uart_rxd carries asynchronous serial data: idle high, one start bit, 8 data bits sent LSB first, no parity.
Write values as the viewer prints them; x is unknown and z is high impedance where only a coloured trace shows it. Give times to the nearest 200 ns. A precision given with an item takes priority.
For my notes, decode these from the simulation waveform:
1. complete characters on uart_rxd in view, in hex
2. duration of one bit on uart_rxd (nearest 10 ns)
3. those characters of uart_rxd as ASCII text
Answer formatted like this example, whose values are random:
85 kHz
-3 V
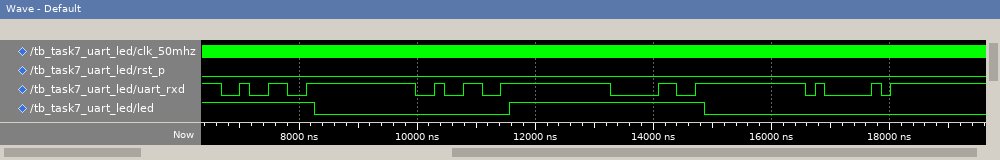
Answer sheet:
32, 32, 30, 41
160 ns
"220A"
